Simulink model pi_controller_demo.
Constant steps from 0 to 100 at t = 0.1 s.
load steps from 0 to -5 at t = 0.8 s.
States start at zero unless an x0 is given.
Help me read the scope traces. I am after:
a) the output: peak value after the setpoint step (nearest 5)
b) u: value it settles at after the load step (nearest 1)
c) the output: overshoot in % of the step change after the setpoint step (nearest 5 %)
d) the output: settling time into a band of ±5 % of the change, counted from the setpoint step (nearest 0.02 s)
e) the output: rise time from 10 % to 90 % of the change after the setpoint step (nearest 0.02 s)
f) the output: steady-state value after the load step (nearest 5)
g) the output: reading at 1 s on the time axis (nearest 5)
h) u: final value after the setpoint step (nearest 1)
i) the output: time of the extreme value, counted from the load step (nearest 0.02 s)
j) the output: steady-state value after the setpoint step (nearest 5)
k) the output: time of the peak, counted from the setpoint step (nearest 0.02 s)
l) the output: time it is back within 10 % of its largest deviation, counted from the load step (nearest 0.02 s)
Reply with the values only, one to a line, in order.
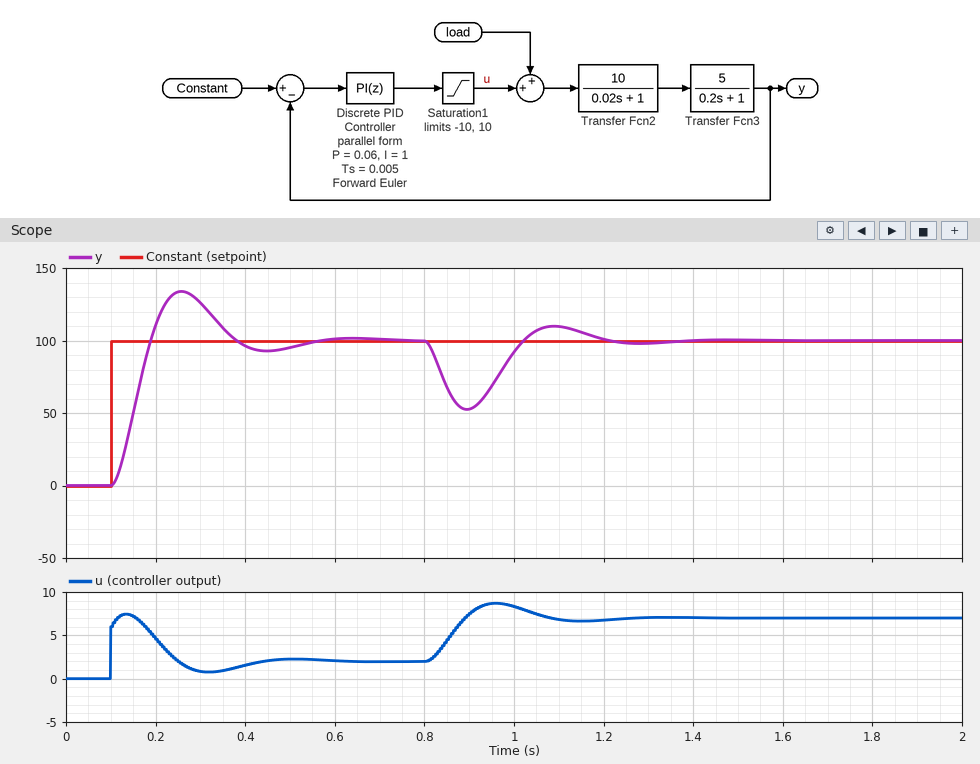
135
7
35 %
0.40 s
0.06 s
100
90
2
0.10 s
100
0.16 s
0.36 s
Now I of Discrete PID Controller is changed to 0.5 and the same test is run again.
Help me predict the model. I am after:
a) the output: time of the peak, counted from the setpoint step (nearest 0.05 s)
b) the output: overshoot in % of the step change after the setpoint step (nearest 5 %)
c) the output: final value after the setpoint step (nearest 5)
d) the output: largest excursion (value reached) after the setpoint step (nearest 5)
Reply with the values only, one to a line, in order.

0.20 s
10 %
100
110
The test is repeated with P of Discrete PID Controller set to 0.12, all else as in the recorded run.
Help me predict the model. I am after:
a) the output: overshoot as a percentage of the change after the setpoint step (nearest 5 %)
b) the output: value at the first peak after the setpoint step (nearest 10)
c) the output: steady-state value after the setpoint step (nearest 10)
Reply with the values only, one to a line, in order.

20 %
120
100
